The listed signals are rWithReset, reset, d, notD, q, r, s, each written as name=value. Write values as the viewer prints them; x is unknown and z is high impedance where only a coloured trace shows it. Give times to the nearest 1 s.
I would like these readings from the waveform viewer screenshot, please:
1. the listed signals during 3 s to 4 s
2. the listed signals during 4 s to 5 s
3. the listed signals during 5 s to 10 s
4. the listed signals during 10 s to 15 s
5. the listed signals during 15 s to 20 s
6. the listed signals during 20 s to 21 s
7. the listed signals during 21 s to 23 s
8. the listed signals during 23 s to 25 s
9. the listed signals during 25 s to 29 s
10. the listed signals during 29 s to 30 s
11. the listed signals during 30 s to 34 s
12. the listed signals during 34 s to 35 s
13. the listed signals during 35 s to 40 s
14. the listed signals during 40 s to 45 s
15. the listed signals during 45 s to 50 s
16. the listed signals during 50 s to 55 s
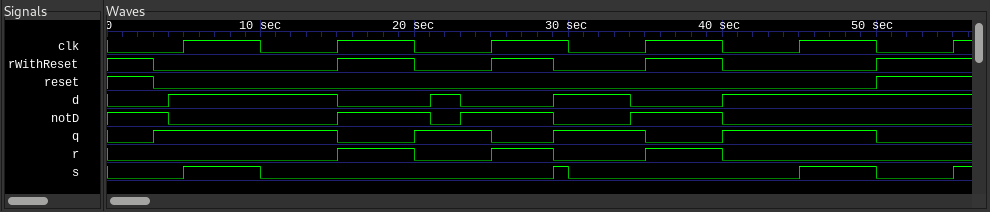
rWithReset=0, reset=0, d=0, notD=1, q=1, r=0, s=0
rWithReset=0, reset=0, d=1, notD=0, q=1, r=0, s=0
rWithReset=0, reset=0, d=1, notD=0, q=1, r=0, s=1
rWithReset=0, reset=0, d=1, notD=0, q=1, r=0, s=0
rWithReset=1, reset=0, d=0, notD=1, q=0, r=1, s=0
rWithReset=0, reset=0, d=0, notD=1, q=1, r=0, s=0
rWithReset=0, reset=0, d=1, notD=0, q=1, r=0, s=0
rWithReset=0, reset=0, d=0, notD=1, q=1, r=0, s=0
rWithReset=1, reset=0, d=0, notD=1, q=0, r=1, s=0
rWithReset=0, reset=0, d=1, notD=0, q=1, r=0, s=1
rWithReset=0, reset=0, d=1, notD=0, q=1, r=0, s=0
rWithReset=0, reset=0, d=0, notD=1, q=1, r=0, s=0
rWithReset=1, reset=0, d=0, notD=1, q=0, r=1, s=0
rWithReset=0, reset=0, d=1, notD=0, q=1, r=0, s=0
rWithReset=0, reset=0, d=1, notD=0, q=1, r=0, s=1
rWithReset=1, reset=1, d=1, notD=0, q=0, r=0, s=0
